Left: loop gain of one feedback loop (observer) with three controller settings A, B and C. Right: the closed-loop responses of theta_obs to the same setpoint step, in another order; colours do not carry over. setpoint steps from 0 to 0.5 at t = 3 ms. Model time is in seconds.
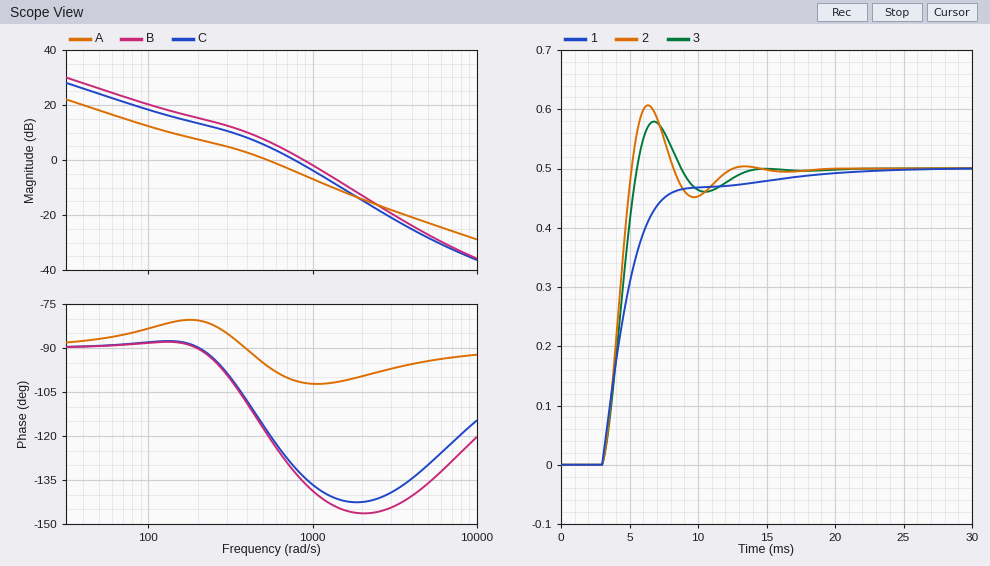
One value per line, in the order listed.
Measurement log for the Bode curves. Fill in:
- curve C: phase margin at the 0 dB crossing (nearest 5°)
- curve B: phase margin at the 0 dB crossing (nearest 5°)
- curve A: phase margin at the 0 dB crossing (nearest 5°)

50°
45°
85°
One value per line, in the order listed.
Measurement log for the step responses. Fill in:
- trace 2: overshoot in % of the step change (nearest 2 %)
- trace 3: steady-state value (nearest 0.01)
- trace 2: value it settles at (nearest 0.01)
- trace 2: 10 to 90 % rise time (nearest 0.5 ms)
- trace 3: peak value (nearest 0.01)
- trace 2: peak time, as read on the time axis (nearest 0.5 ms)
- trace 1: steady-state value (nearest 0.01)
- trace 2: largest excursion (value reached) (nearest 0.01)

22 %
0.50
0.50
1.5 ms
0.58
6.5 ms
0.50
0.61
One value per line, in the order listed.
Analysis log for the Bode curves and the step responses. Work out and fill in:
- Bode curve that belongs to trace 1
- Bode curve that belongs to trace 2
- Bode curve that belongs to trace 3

A
B
C
